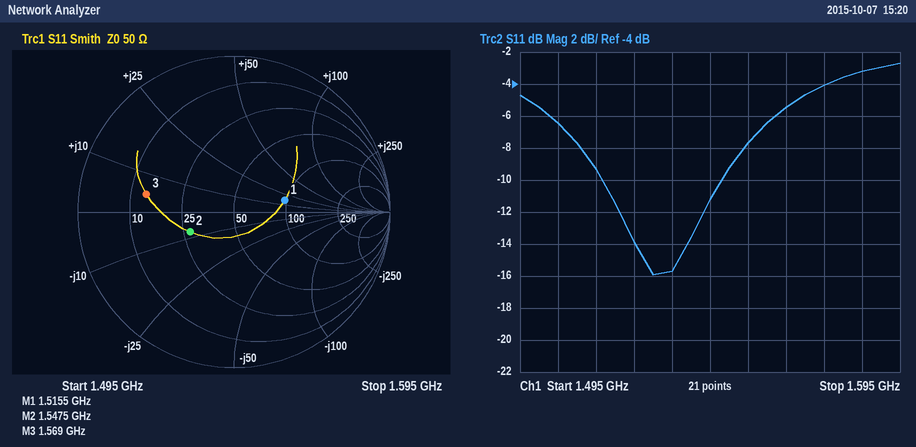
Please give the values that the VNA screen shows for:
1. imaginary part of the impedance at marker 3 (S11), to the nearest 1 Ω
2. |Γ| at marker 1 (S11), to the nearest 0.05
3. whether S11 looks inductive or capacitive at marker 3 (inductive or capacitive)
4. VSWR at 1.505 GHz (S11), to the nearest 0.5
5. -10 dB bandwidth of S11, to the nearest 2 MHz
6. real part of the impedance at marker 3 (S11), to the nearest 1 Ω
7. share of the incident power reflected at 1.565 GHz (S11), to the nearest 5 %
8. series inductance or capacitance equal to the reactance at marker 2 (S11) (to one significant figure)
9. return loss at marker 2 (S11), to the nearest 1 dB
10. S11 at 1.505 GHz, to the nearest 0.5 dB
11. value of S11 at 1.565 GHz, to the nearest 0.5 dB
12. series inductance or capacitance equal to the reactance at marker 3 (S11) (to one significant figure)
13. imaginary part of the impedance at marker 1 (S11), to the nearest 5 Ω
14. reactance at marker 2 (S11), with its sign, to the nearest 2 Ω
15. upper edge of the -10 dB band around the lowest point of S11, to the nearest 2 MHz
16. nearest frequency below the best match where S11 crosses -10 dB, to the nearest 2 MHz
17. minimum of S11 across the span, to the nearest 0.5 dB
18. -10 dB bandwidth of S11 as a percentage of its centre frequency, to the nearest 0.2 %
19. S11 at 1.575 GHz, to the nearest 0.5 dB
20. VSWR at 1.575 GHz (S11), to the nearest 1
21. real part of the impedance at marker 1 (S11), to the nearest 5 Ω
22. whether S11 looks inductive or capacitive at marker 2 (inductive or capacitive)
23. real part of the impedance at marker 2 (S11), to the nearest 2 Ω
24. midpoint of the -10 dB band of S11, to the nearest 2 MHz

+5 Ω
0.35
inductive
3.0
32 MHz
14 Ω
30 %
10 pF
10 dB
-6.5 dB
-5.5 dB
500 pH
+15 Ω
-8 Ω
1.548 GHz
1.516 GHz
-16.0 dB
2.0 %
-4.0 dB
4
95 Ω
capacitive
28 Ω
1.532 GHz
